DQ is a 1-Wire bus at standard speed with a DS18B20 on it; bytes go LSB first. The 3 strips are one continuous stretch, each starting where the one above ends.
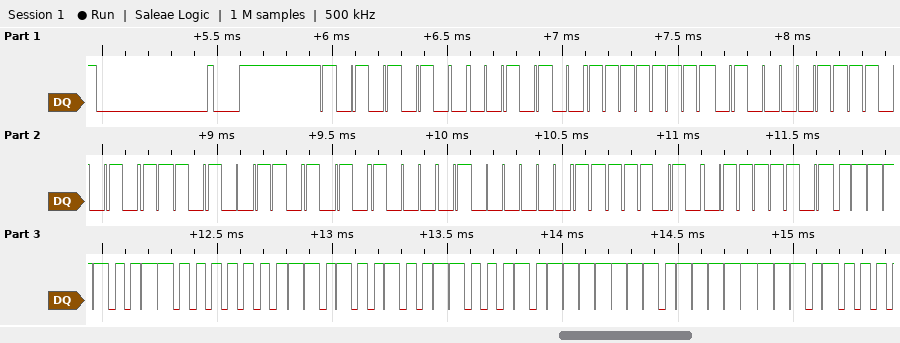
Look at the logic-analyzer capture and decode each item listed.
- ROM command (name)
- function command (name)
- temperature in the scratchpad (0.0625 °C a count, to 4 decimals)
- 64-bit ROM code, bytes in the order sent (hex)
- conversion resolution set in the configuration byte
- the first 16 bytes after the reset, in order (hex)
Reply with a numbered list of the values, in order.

1. Match ROM
2. Read Scratchpad
3. 25.8750 °C
4. 28 FF C2 D3 65 15 02 5F
5. 12 bits
6. 55 28 FF C2 D3 65 15 02 5F BE 9E 01 4B 46 7F FF
